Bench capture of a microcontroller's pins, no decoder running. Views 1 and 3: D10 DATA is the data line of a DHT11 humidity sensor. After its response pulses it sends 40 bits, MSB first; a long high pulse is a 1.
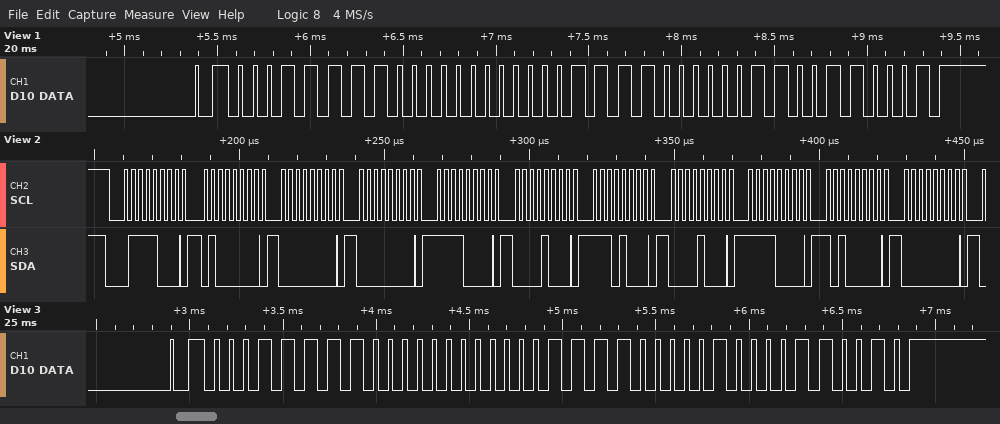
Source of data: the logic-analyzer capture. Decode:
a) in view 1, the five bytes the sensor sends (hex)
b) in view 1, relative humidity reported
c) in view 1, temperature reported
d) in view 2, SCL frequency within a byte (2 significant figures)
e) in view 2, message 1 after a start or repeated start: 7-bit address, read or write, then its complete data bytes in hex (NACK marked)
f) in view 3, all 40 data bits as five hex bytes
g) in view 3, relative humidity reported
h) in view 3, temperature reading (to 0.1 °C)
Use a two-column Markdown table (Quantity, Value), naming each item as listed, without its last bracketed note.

| Quantity | Value |
|---|---|
| in view 1, the five bytes the sensor sends | 1F 00 0F 03 31 |
| in view 1, relative humidity reported | 31 % |
| in view 1, temperature reported | 15.3 °C |
| in view 2, SCL frequency within a byte | 400 kHz |
| in view 2, message 1 after a start or repeated start: 7-bit address, read or write, then its complete data bytes in hex | 0x3C write: 40 00 00 F0 08 E8 08 F0 A0 00 |
| in view 3, all 40 data bits as five hex bytes | 1F 00 0F 04 32 |
| in view 3, relative humidity reported | 31 % |
| in view 3, temperature reading | 15.4 °C |
